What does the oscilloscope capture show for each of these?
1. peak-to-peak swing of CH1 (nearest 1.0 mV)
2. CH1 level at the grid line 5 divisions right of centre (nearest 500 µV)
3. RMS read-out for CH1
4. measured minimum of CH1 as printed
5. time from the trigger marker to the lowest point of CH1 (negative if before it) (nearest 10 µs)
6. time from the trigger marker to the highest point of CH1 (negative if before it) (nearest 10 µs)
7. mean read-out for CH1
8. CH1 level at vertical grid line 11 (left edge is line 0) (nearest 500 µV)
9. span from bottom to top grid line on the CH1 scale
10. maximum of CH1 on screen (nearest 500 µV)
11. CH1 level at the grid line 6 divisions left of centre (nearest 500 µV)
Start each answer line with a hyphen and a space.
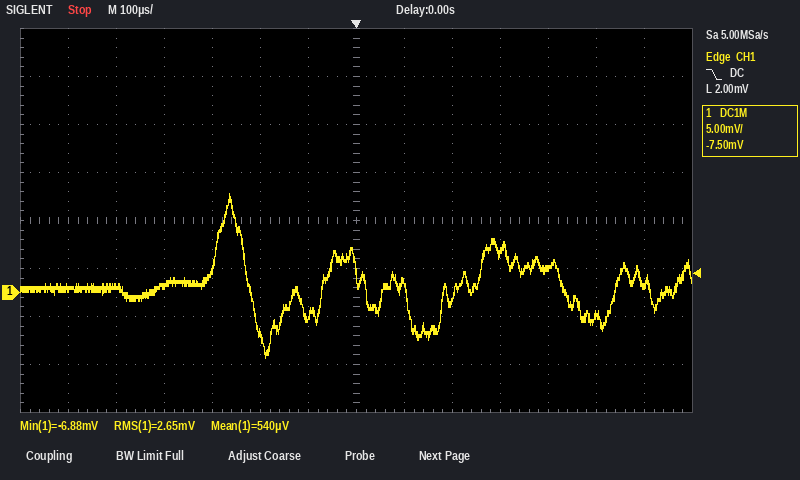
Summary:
- 17.0 mV
- -2.5 mV
- 2.65 mV
- -6.88 mV
- -190 µs
- -260 µs
- 540 µV
- 2.5 mV
- 40 mV
- 10.5 mV
- 500 µV
